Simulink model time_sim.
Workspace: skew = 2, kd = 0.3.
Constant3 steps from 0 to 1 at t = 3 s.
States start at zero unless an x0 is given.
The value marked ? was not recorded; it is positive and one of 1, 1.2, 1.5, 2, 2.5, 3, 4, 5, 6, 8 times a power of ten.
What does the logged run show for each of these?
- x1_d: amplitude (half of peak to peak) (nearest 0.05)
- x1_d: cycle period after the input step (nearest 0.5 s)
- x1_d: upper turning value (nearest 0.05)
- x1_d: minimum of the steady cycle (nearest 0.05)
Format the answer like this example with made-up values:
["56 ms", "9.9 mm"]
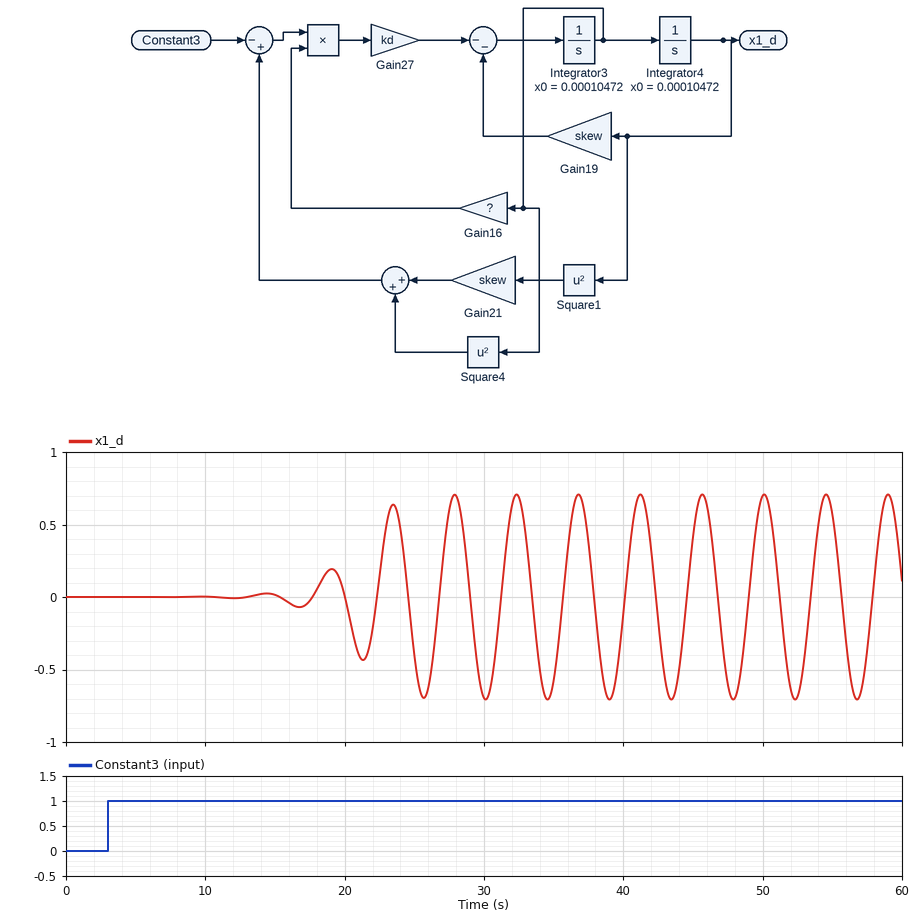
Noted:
["0.70", "4.5 s", "0.70", "-0.70"]
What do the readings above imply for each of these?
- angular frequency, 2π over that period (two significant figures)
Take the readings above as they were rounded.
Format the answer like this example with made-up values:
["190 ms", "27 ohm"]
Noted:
["1.4 rad/s"]
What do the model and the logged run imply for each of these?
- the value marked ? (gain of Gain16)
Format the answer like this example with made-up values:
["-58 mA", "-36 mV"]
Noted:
["3"]
